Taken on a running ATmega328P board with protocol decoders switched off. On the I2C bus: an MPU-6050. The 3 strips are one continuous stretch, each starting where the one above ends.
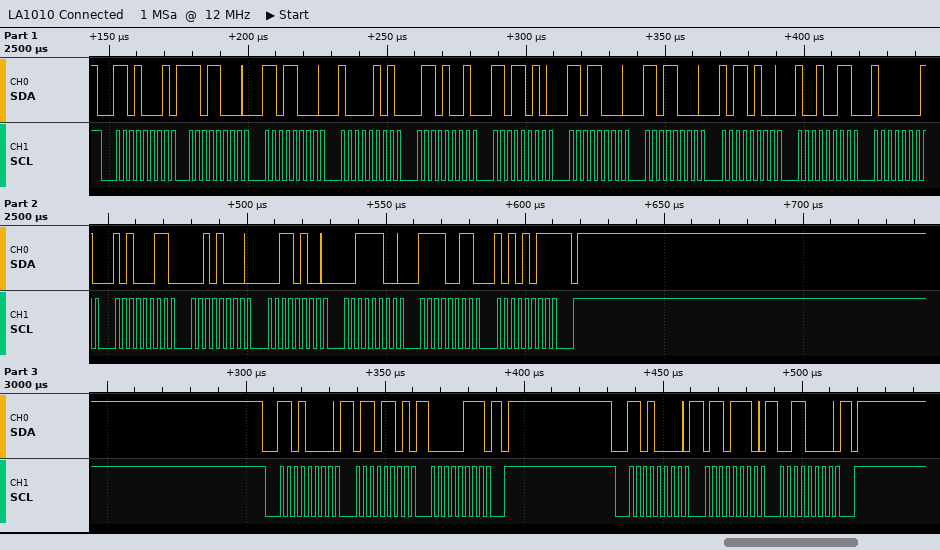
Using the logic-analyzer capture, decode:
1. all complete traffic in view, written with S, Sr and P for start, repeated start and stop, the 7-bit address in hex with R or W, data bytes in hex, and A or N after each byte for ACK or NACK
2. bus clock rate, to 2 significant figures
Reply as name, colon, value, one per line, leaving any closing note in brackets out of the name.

all complete traffic in view, written with S, Sr and P for start, repeated start and stop, the 7-bit address in hex with R or W, data bytes in hex, and A or N after each byte for ACK or NACK: S 68R A D8 A D8 A 85 A 69 A DA A D8 A D8 A B4 A 93 A 81 A A3 A 28 A 34 A 3C A F3 A AB N P S 68W A 6D A 07 A P S 68W A 6E A 30 A P
bus clock rate, to 2 significant figures: 400 kHz
